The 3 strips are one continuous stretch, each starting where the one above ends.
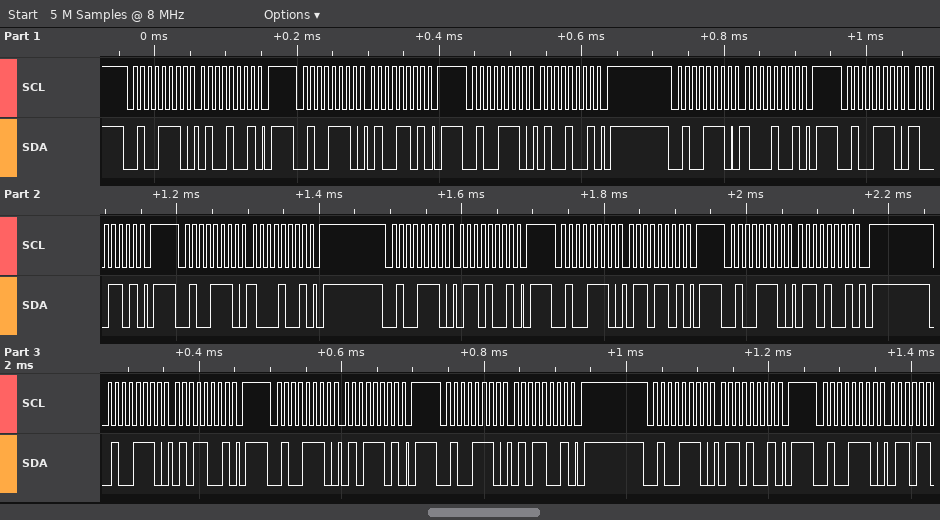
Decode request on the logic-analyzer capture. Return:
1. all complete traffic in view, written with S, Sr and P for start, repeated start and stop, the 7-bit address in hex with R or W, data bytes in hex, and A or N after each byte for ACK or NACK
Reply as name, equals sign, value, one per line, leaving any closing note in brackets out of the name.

all complete traffic in view, written with S, Sr and P for start, repeated start and stop, the 7-bit address in hex with R or W, data bytes in hex, and A or N after each byte for ACK or NACK = S 27W A 49 A P S 27W A 4D A P S 27W A 49 A P S 27W A 89 A P S 27W A 8D A P S 27W A 89 A P S 27W A 69 A P S 27W A 6D A P S 27W A 69 A P S 27W A 59 A P S 27W A 5D A P S 27W A 59 A P S 27W A 69 A P S 27W A
